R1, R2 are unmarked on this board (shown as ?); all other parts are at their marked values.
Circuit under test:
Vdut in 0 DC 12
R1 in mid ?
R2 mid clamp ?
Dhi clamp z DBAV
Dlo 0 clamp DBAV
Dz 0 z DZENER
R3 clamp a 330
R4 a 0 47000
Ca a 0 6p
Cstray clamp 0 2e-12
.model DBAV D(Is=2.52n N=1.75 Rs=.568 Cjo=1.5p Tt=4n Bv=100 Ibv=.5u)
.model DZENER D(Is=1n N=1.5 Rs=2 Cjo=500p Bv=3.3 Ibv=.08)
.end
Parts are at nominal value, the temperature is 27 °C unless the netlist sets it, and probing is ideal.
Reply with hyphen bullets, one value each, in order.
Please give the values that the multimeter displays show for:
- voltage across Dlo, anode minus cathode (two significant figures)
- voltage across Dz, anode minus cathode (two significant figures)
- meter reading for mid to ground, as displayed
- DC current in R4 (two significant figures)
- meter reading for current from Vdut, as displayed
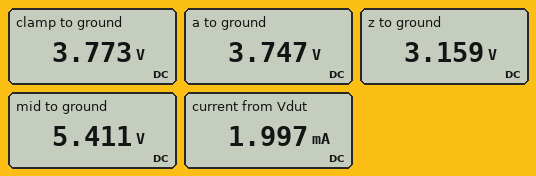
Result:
- -3.8 V
- -3.2 V
- 5.411 V
- 80 µA
- 1.997 mA
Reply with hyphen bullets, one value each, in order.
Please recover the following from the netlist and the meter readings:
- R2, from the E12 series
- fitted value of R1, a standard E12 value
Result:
- 820 Ω
- 3.3 kΩ
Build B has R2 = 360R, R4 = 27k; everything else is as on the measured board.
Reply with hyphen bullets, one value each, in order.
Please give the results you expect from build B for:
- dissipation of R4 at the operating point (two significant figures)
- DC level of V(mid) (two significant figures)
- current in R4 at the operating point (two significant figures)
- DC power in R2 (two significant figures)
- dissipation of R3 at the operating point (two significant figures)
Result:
- 520 µW
- 4.6 V
- 140 µA
- 1.8 mW
- 6.3 µW
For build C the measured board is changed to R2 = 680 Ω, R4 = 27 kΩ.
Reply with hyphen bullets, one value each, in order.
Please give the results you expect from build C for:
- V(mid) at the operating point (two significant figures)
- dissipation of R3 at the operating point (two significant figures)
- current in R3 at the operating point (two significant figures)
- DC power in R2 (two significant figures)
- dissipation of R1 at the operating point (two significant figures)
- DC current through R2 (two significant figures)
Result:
- 5.2 V
- 6.3 µW
- 140 µA
- 2.9 mW
- 14 mW
- 2.1 mA
